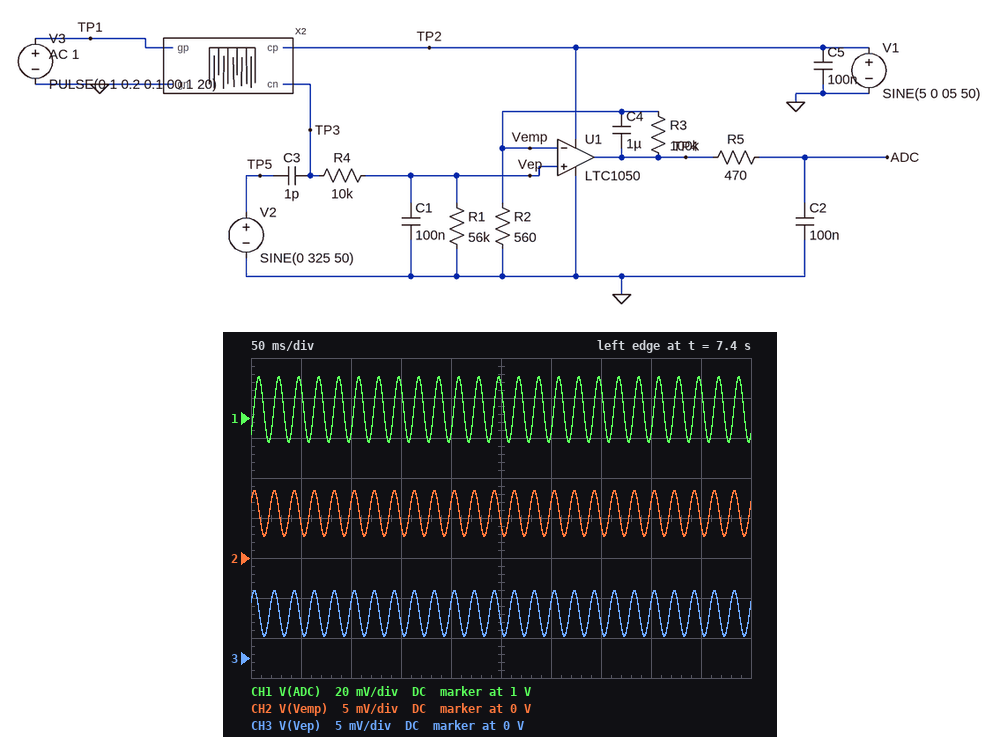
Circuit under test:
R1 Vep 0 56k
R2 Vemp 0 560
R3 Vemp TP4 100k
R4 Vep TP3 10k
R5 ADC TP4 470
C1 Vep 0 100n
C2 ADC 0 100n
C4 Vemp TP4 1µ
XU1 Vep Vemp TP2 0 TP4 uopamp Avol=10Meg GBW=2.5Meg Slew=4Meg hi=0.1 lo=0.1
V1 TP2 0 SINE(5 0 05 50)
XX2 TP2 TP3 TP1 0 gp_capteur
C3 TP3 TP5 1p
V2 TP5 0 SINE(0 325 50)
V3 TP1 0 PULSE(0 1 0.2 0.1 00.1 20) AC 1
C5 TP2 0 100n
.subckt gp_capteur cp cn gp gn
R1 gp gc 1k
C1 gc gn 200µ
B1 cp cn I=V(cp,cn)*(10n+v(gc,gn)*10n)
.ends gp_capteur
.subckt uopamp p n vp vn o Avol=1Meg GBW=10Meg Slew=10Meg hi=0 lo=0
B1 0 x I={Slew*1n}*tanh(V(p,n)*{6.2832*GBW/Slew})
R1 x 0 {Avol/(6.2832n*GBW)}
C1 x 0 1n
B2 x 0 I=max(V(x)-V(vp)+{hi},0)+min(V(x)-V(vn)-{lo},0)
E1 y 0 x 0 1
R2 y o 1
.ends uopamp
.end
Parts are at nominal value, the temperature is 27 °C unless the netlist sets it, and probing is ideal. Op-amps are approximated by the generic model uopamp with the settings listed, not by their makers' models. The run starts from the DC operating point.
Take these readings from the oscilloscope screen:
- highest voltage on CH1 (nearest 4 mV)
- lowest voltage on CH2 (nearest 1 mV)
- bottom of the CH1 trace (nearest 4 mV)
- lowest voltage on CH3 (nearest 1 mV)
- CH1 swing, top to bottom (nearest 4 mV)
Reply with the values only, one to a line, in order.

1.020 V
3 mV
988 mV
3 mV
32 mV
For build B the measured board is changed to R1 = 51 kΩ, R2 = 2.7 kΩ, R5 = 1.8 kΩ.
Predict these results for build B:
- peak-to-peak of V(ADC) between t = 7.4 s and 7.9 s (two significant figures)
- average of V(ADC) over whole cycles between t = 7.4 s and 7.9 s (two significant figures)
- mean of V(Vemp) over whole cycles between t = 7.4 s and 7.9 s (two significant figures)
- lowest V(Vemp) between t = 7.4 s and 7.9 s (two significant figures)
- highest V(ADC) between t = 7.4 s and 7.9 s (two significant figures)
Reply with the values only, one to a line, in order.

8.6 mV
190 mV
5.1 mV
2.3 mV
200 mV
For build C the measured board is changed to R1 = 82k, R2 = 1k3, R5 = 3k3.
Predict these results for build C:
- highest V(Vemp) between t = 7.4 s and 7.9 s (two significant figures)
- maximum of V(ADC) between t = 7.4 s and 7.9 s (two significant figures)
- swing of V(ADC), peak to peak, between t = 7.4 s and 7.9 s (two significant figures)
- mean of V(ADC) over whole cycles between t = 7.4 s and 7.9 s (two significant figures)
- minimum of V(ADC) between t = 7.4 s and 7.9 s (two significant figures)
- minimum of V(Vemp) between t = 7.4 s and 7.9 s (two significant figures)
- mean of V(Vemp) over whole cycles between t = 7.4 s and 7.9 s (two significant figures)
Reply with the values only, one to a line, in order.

11 mV
650 mV
16 mV
640 mV
630 mV
5.2 mV
8.2 mV
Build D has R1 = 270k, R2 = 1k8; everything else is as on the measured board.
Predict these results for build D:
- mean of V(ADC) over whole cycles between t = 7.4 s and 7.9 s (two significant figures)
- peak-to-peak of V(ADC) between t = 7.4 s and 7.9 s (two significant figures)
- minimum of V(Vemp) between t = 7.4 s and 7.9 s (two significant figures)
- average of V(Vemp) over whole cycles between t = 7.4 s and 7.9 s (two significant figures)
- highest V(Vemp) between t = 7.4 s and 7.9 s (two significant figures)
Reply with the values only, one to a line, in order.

1.5 V
13 mV
24 mV
27 mV
30 mV
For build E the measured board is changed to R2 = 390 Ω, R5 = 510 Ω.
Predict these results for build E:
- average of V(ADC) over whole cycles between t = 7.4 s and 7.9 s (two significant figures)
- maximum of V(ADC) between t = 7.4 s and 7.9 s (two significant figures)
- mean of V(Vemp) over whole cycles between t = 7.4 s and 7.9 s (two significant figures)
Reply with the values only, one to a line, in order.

1.4 V
1.5 V
5.6 mV
